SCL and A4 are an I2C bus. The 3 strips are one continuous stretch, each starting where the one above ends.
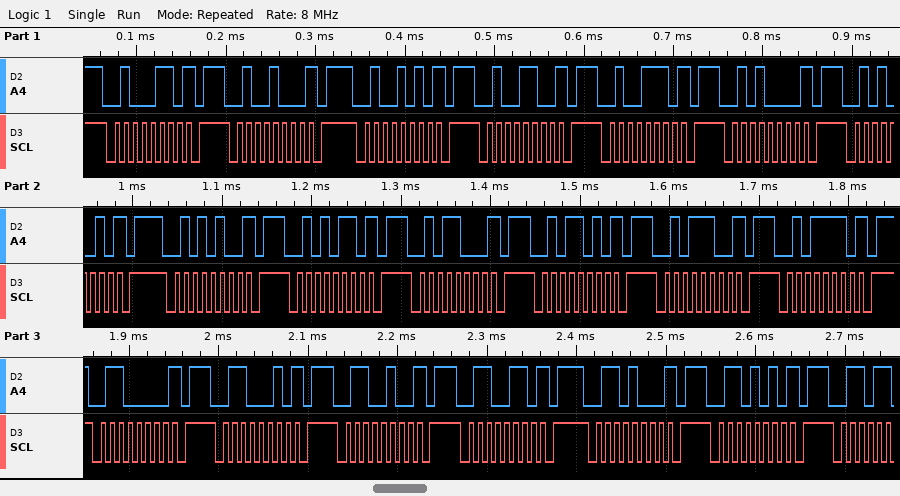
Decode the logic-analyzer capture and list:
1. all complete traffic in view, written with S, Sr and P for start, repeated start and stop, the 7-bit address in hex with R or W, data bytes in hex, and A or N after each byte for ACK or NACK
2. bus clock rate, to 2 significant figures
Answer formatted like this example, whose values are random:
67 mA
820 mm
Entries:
S 23W N P S 24W N P S 25W N P S 26W N P S 27W N P S 28W N P S 29W N P S 2AW N P S 2BW N P S 2CW N P S 2DW N P S 2EW N P S 2FW N P S 30W N P S 31W N P S 32W N P S 33W N P S 34W N P S 35W N P
100 kHz
